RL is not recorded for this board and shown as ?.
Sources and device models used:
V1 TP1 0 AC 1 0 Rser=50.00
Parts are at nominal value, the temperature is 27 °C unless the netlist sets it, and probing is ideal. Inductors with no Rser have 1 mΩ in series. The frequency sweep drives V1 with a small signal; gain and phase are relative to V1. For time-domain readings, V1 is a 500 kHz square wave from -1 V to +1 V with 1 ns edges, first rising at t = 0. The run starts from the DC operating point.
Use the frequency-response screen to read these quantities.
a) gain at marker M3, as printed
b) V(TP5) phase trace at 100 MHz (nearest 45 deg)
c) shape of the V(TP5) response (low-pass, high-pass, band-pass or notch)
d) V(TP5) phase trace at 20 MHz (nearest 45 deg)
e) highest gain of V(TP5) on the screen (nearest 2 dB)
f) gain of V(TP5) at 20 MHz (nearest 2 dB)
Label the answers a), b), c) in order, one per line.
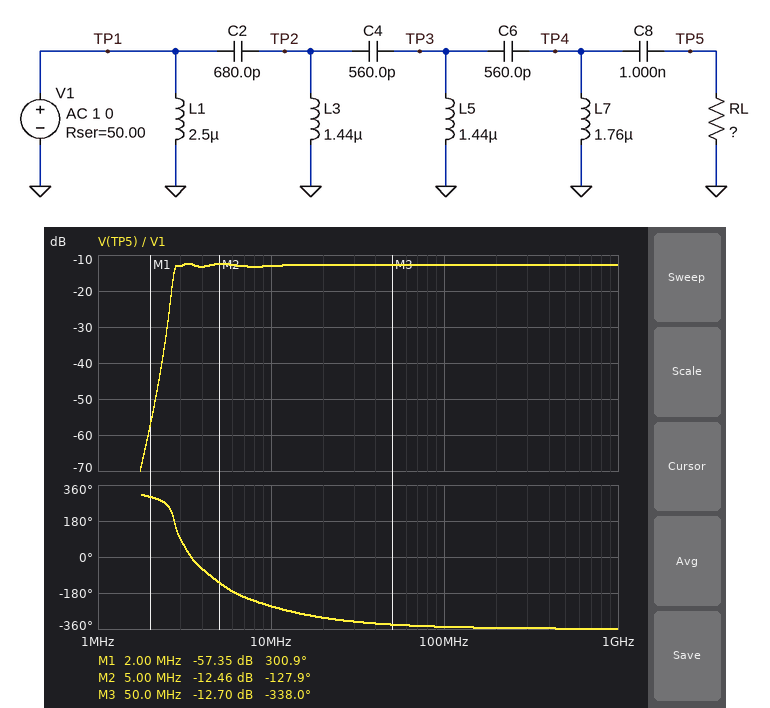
a) -12.70 dB
b) -360 deg
c) high-pass
d) -315 deg
e) -12 dB
f) -12 dB
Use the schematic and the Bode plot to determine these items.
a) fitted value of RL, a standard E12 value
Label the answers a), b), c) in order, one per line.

a) 15 Ω
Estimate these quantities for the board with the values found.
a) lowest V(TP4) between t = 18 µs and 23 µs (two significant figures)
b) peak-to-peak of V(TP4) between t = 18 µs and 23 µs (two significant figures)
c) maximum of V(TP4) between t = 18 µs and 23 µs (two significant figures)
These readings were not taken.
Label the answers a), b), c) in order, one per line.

a) -370 mV
b) 740 mV
c) 370 mV
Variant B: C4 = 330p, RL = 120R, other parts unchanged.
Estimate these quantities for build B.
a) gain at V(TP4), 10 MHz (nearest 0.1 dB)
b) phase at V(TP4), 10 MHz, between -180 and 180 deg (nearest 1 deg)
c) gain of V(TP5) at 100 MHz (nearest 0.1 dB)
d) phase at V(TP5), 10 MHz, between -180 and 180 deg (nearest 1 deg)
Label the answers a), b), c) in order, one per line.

a) -2.4 dB
b) 115 deg
c) -3.0 dB
d) 123 deg
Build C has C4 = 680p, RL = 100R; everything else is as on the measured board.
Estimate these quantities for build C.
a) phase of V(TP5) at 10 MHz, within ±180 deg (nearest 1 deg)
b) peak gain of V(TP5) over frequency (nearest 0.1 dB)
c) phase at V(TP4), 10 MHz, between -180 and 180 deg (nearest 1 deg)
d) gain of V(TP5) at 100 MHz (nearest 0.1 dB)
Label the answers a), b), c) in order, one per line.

a) 104 deg
b) -3.2 dB
c) 95 deg
d) -3.5 dB
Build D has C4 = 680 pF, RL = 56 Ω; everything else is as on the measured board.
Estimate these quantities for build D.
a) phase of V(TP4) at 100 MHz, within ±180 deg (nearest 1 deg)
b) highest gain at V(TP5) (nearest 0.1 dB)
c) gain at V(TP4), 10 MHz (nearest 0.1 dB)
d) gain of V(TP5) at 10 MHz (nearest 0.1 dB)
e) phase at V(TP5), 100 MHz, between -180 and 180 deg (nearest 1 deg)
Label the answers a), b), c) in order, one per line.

a) 9 deg
b) -5.5 dB
c) -5.3 dB
d) -5.6 dB
e) 11 deg
